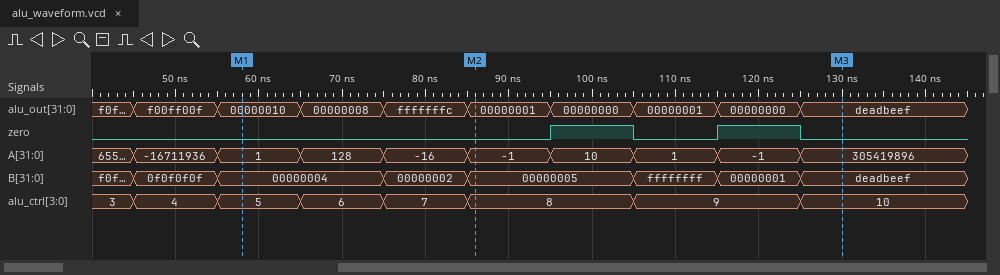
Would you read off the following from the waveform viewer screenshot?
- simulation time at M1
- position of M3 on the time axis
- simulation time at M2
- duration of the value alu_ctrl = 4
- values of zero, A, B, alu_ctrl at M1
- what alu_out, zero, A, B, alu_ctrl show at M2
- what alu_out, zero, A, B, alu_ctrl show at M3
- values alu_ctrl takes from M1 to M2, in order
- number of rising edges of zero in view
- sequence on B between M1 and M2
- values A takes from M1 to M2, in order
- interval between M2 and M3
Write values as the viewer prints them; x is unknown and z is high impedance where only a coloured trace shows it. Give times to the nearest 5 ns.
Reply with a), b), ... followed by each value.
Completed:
a) 60 ns
b) 130 ns
c) 85 ns
d) 10 ns
e) zero=0, A=1, B=00000004, alu_ctrl=5
f) alu_out=00000001, zero=0, A=-1, B=00000005, alu_ctrl=8
g) alu_out=deadbeef, zero=0, A=305419896, B=deadbeef, alu_ctrl=10
h) 5, 6, 7, 8
i) 2
j) 00000004, 00000002, 00000005
k) 1, 128, -16, -1
l) 45 ns
